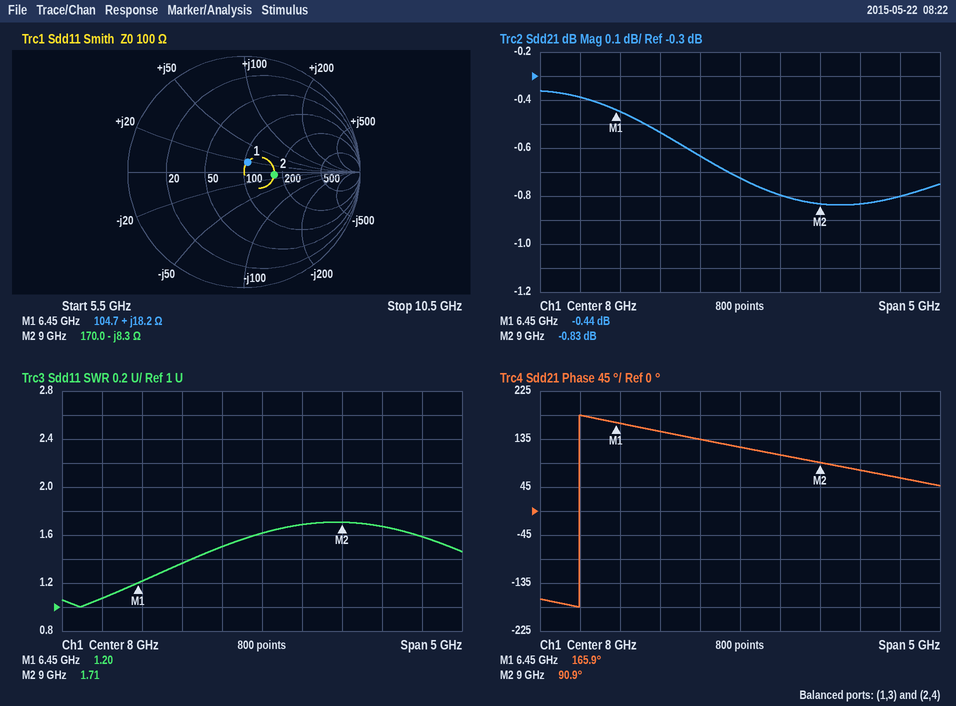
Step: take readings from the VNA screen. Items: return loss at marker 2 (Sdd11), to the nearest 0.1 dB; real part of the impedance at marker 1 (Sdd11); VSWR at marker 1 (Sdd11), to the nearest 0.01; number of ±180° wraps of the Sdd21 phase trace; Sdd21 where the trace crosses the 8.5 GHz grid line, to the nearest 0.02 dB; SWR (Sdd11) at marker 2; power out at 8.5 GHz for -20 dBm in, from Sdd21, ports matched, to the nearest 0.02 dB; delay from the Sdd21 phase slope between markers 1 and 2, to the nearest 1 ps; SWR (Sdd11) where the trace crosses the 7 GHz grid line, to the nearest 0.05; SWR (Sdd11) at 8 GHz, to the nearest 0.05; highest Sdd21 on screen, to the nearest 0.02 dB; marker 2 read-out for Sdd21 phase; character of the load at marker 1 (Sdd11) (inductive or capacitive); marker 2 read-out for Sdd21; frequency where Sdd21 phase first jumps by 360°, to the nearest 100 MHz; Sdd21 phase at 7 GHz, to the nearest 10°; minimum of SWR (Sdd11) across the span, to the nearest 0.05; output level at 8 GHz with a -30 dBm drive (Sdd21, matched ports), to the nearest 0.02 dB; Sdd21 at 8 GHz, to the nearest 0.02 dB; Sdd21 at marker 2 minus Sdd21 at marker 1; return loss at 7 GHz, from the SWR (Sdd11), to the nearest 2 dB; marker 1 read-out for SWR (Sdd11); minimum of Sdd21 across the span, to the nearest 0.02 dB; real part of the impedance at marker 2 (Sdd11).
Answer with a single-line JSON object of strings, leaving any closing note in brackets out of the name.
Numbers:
{"return loss at marker 2 (Sdd11), to the nearest 0.1 dB": "11.7 dB", "real part of the impedance at marker 1": "104.7 Ω", "VSWR at marker 1 (Sdd11), to the nearest 0.01": "1.20", "number of ±180° wraps of the Sdd21 phase trace": "1", "Sdd21 where the trace crosses the 8.5 GHz grid line, to the nearest 0.02 dB": "-0.80 dB", "SWR (Sdd11) at marker 2": "1.71", "power out at 8.5 GHz for -20 dBm in, from Sdd21, ports matched, to the nearest 0.02 dB": "-20.80 dBm", "delay from the Sdd21 phase slope between markers 1 and 2, to the nearest 1 ps": "82 ps", "SWR (Sdd11) where the trace crosses the 7 GHz grid line, to the nearest 0.05": "1.35", "SWR (Sdd11) at 8 GHz, to the nearest 0.05": "1.60", "highest Sdd21 on screen, to the nearest 0.02 dB": "-0.36 dB", "marker 2 read-out for Sdd21 phase": "90.9°", "character of the load at marker 1 (Sdd11)": "inductive", "marker 2 read-out for Sdd21": "-0.83 dB", "frequency where Sdd21 phase first jumps by 360°, to the nearest 100 MHz": "6.0 GHz", "Sdd21 phase at 7 GHz, to the nearest 10°": "150°", "minimum of SWR (Sdd11) across the span, to the nearest 0.05": "1.00", "output level at 8 GHz with a -30 dBm drive (Sdd21, matched ports), to the nearest 0.02 dB": "-30.72 dBm", "Sdd21 at 8 GHz, to the nearest 0.02 dB": "-0.72 dB", "Sdd21 at marker 2 minus Sdd21 at marker 1": "-0.39 dB", "return loss at 7 GHz, from the SWR (Sdd11), to the nearest 2 dB": "16 dB", "marker 1 read-out for SWR": "1.20", "minimum of Sdd21 across the span, to the nearest 0.02 dB": "-0.84 dB", "real part of the impedance at marker 2": "170.0 Ω"}
